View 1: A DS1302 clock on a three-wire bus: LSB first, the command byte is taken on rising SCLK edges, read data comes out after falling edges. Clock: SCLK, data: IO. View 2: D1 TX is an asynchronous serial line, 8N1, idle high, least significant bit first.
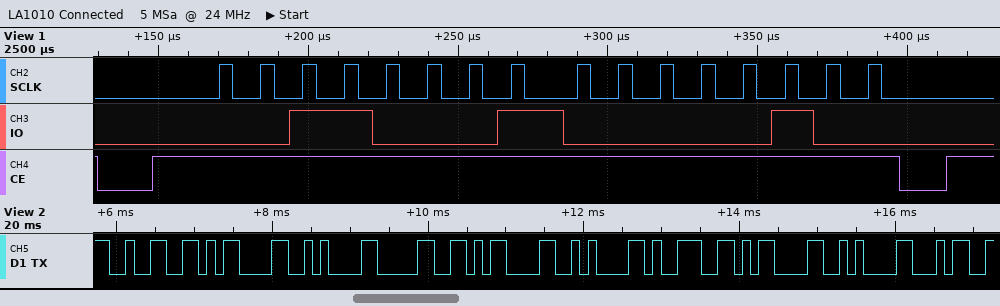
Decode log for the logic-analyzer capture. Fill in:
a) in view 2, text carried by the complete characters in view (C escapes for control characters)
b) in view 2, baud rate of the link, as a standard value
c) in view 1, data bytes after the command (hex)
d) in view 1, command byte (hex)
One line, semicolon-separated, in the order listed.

"2\r\n0\r\n9\r\n4"; 9600 baud; 20; 0x8C
